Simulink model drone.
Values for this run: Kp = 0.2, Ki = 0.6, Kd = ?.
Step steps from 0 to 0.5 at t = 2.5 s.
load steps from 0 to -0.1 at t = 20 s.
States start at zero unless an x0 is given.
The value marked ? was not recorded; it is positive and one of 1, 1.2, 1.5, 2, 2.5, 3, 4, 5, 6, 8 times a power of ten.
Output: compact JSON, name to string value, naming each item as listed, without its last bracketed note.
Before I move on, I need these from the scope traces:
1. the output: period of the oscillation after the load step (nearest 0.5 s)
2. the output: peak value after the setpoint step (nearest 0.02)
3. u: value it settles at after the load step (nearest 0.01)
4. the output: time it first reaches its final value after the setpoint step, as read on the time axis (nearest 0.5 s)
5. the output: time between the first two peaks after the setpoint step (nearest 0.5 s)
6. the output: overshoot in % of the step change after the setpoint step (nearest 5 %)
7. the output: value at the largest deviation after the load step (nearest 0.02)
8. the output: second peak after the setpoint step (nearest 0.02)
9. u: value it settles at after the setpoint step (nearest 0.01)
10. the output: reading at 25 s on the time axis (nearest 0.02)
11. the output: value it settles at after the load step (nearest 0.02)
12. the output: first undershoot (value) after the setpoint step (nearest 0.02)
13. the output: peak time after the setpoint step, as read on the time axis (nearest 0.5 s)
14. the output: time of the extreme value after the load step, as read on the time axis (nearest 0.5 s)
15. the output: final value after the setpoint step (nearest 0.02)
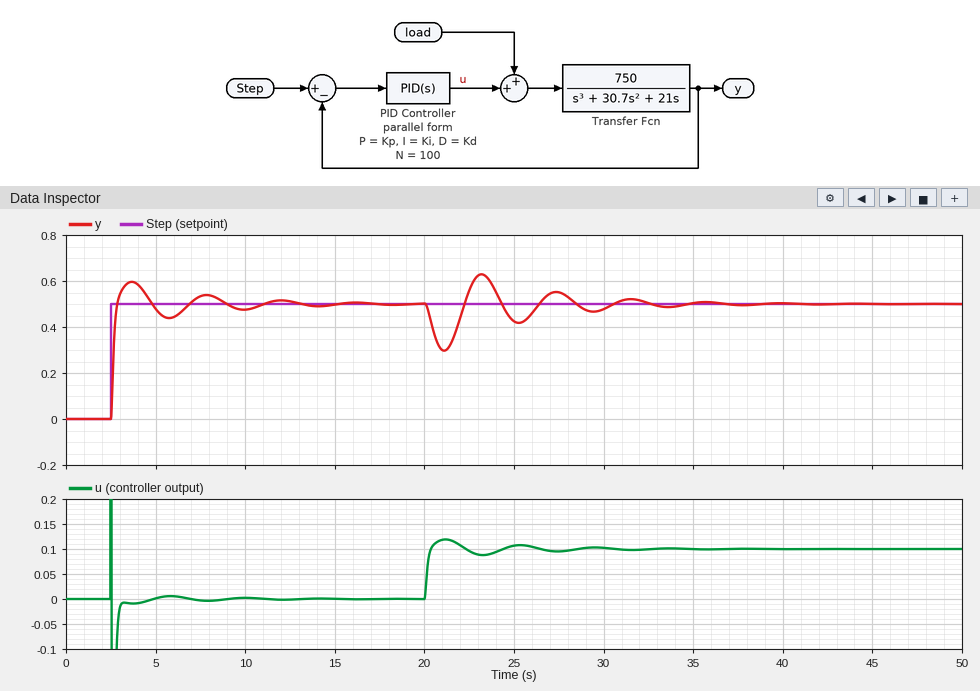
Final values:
{"the output: period of the oscillation after the load step": "4.0 s", "the output: peak value after the setpoint step": "0.60", "u: value it settles at after the load step": "0.10", "the output: time it first reaches its final value after the setpoint step, as read on the time axis": "3.0 s", "the output: time between the first two peaks after the setpoint step": "4.0 s", "the output: overshoot in % of the step change after the setpoint step": "20 %", "the output: value at the largest deviation after the load step": "0.30", "the output: second peak after the setpoint step": "0.54", "u: value it settles at after the setpoint step": "0.00", "the output: reading at 25 s on the time axis": "0.42", "the output: value it settles at after the load step": "0.50", "the output: first undershoot (value) after the setpoint step": "0.44", "the output: peak time after the setpoint step, as read on the time axis": "3.5 s", "the output: time of the extreme value after the load step, as read on the time axis": "21.0 s", "the output: final value after the setpoint step": "0.50"}
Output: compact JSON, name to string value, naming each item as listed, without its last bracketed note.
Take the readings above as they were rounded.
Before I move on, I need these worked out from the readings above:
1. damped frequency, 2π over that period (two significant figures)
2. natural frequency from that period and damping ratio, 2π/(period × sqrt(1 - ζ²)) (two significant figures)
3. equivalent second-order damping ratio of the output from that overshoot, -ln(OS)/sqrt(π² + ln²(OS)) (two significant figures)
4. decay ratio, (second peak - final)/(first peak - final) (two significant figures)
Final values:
{"damped frequency, 2π over that period": "1.6 rad/s", "natural frequency from that period and damping ratio, 2π/(period × sqrt(1 - ζ²))": "1.8 rad/s", "equivalent second-order damping ratio of the output from that overshoot, -ln(OS)/sqrt(π² + ln²(OS))": "0.46", "decay ratio, (second peak - final)/(first peak - final)": "0.40"}
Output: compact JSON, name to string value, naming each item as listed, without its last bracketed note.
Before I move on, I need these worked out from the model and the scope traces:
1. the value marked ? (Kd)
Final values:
{"the value marked ?": "0.25"}
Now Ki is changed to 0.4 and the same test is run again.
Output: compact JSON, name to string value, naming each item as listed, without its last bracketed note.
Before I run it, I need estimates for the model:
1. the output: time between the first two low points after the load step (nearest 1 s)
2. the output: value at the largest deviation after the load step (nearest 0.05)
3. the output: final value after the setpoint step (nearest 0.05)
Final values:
{"the output: time between the first two low points after the load step": "5 s", "the output: value at the largest deviation after the load step": "0.25", "the output: final value after the setpoint step": "0.50"}
